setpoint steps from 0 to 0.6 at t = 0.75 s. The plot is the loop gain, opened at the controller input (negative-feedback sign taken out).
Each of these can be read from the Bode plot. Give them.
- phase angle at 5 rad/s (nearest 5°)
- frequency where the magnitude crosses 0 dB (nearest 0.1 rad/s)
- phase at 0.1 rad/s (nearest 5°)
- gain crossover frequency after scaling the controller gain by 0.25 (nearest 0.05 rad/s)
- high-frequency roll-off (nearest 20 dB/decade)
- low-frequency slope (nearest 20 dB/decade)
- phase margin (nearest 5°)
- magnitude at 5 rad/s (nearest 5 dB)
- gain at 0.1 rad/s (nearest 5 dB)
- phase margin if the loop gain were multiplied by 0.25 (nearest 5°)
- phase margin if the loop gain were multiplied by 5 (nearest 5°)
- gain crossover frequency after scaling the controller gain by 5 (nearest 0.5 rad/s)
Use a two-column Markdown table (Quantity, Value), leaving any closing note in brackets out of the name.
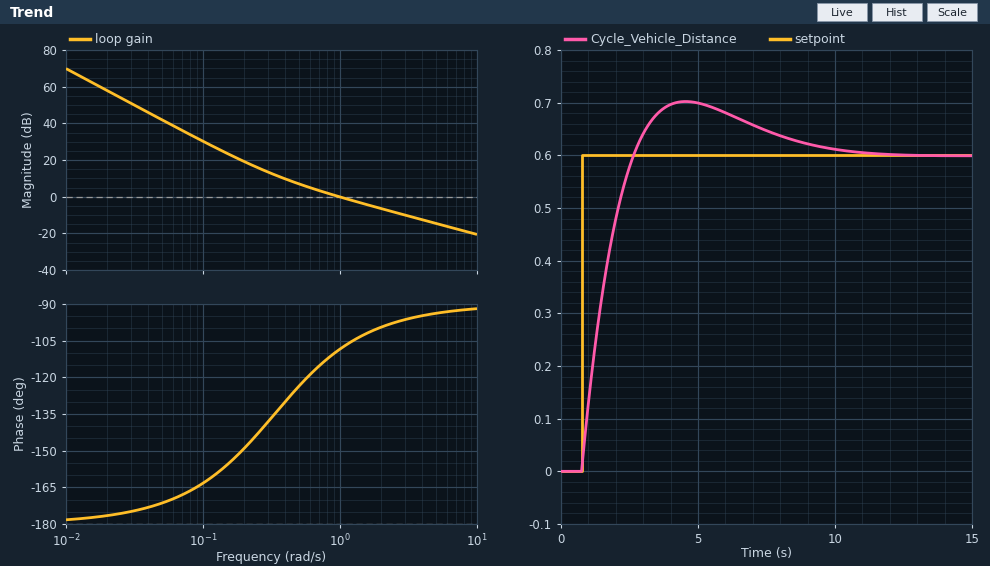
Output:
| Quantity | Value |
|---|---|
| phase angle at 5 rad/s | -95° |
| frequency where the magnitude crosses 0 dB | 1.0 rad/s |
| phase at 0.1 rad/s | -165° |
| gain crossover frequency after scaling the controller gain by 0.25 | 0.35 rad/s |
| high-frequency roll-off | -20 dB/decade |
| low-frequency slope | -40 dB/decade |
| phase margin | 70° |
| magnitude at 5 rad/s | -15 dB |
| gain at 0.1 rad/s | 30 dB |
| phase margin if the loop gain were multiplied by 0.25 | 45° |
| phase margin if the loop gain were multiplied by 5 | 85° |
| gain crossover frequency after scaling the controller gain by 5 | 4.5 rad/s |
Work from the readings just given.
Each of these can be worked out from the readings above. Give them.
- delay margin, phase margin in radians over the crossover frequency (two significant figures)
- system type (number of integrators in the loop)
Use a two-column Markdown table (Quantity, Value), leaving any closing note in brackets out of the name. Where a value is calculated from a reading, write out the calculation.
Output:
| Quantity | Value |
|---|---|
| delay margin, phase margin in radians over the crossover frequency | 70 × π / 180 / 1 = 1.2 s |
| system type | 2 |
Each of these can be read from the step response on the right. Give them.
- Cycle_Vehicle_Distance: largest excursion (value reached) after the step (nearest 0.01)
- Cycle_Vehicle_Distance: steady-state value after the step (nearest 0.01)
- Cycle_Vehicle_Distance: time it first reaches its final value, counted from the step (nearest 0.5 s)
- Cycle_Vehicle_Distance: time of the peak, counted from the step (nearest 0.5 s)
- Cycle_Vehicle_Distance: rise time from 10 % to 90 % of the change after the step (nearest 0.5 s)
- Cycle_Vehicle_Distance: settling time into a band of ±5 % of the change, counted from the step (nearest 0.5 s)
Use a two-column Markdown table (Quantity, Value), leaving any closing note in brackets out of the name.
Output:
| Quantity | Value |
|---|---|
| Cycle_Vehicle_Distance: largest excursion (value reached) after the step | 0.70 |
| Cycle_Vehicle_Distance: steady-state value after the step | 0.60 |
| Cycle_Vehicle_Distance: time it first reaches its final value, counted from the step | 2.0 s |
| Cycle_Vehicle_Distance: time of the peak, counted from the step | 4.0 s |
| Cycle_Vehicle_Distance: rise time from 10 % to 90 % of the change after the step | 1.5 s |
| Cycle_Vehicle_Distance: settling time into a band of ±5 % of the change, counted from the step | 7.5 s |
